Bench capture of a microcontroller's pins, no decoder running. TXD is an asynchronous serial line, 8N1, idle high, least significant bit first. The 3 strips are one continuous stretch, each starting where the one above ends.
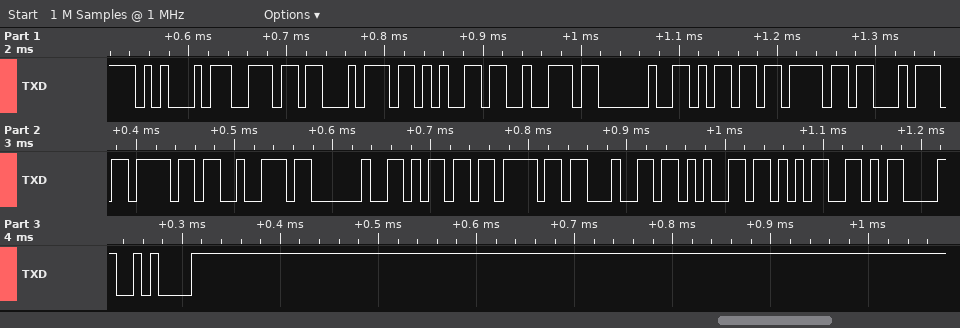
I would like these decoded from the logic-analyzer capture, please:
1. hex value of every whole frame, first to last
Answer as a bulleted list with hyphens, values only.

- 45 6E 74 65 72 20 6D 6F 74 6F 72 20 6D 6F 64 65 35 0D 0A
